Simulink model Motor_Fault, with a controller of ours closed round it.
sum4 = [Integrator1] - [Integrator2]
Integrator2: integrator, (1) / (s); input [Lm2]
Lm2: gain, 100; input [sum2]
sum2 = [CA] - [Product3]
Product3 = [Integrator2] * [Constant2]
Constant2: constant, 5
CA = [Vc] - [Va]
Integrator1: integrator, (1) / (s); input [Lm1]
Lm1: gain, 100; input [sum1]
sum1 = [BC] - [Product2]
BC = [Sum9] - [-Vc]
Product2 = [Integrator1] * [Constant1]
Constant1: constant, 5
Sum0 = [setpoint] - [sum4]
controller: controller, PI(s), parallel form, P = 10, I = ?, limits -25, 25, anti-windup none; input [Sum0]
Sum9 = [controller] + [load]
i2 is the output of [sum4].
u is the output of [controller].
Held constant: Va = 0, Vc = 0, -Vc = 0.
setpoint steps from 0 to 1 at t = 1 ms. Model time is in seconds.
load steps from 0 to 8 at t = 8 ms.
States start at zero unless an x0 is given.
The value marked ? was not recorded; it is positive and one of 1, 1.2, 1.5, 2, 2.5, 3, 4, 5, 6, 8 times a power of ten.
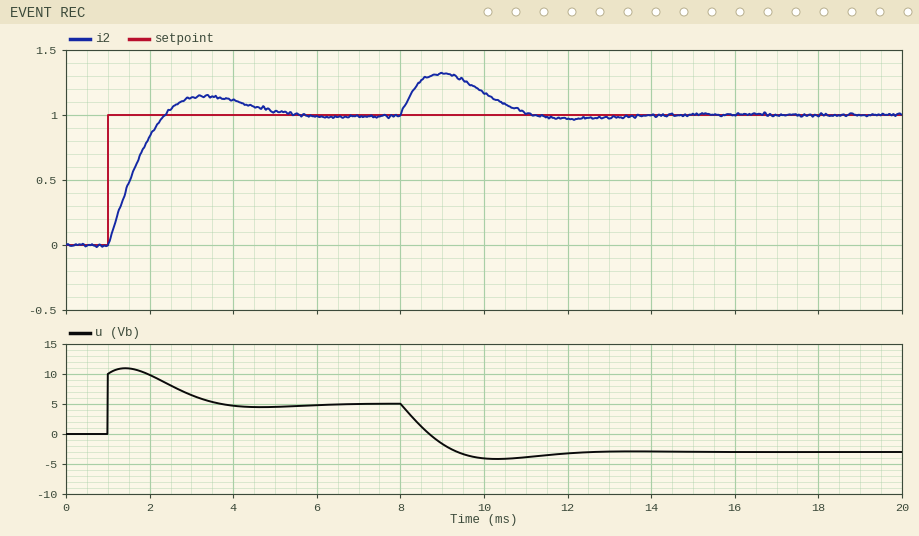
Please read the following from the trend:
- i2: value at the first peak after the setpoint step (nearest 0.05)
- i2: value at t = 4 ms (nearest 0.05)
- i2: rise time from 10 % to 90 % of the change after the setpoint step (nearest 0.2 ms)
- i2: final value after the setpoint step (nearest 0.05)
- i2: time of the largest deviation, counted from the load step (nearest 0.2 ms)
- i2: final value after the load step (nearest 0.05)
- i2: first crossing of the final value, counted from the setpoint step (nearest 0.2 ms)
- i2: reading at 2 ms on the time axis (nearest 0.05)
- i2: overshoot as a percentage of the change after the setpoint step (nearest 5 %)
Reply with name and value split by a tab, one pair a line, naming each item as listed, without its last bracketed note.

i2: value at the first peak after the setpoint step	1.15
i2: value at t = 4 ms	1.10
i2: rise time from 10 % to 90 % of the change after the setpoint step	1.0 ms
i2: final value after the setpoint step	1.00
i2: time of the largest deviation, counted from the load step	1.0 ms
i2: final value after the load step	1.00
i2: first crossing of the final value, counted from the setpoint step	1.4 ms
i2: reading at 2 ms on the time axis	0.85
i2: overshoot as a percentage of the change after the setpoint step	15 %
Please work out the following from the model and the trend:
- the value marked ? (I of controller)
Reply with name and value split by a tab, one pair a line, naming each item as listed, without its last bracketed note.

the value marked ?	15000
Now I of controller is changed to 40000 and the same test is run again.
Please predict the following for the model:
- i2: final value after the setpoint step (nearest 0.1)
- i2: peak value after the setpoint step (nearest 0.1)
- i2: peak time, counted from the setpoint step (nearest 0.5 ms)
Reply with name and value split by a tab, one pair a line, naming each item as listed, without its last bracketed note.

i2: final value after the setpoint step	1.0
i2: peak value after the setpoint step	1.3
i2: peak time, counted from the setpoint step	1.5 ms
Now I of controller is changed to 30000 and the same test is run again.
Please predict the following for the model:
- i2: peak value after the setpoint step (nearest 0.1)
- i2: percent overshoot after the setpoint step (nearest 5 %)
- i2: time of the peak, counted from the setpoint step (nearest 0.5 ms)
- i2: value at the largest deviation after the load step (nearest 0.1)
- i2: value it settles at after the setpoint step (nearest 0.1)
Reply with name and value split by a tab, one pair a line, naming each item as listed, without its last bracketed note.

i2: peak value after the setpoint step	1.3
i2: percent overshoot after the setpoint step	25 %
i2: time of the peak, counted from the setpoint step	1.5 ms
i2: value at the largest deviation after the load step	1.3
i2: value it settles at after the setpoint step	1.0
